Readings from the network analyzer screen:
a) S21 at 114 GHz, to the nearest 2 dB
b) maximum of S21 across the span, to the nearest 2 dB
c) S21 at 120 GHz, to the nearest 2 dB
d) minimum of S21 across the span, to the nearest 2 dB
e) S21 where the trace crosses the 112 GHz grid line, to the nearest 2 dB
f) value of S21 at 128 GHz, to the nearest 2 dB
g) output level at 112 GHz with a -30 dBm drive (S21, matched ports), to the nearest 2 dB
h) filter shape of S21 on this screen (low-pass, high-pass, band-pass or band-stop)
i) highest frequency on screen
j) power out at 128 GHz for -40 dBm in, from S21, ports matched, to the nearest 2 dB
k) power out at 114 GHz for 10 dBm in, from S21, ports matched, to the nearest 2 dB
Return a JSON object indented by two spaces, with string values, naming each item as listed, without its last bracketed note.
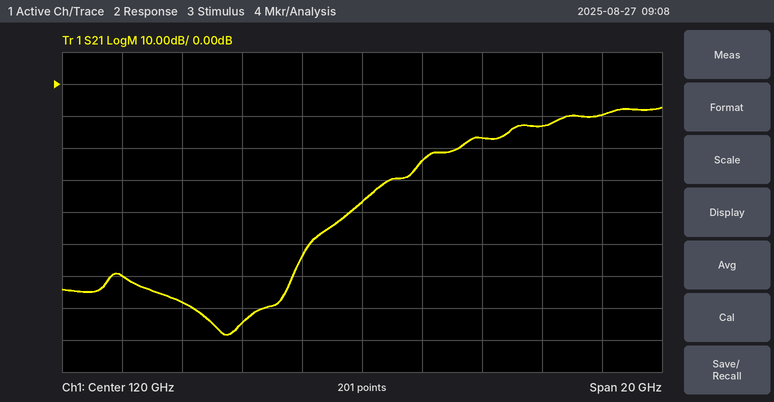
{
  "S21 at 114 GHz, to the nearest 2 dB": "-68 dB",
  "maximum of S21 across the span, to the nearest 2 dB": "-8 dB",
  "S21 at 120 GHz, to the nearest 2 dB": "-36 dB",
  "minimum of S21 across the span, to the nearest 2 dB": "-78 dB",
  "S21 where the trace crosses the 112 GHz grid line, to the nearest 2 dB": "-60 dB",
  "value of S21 at 128 GHz, to the nearest 2 dB": "-10 dB",
  "output level at 112 GHz with a -30 dBm drive (S21, matched ports), to the nearest 2 dB": "-90 dBm",
  "filter shape of S21 on this screen": "high-pass",
  "highest frequency on screen": "130 GHz",
  "power out at 128 GHz for -40 dBm in, from S21, ports matched, to the nearest 2 dB": "-50 dBm",
  "power out at 114 GHz for 10 dBm in, from S21, ports matched, to the nearest 2 dB": "-58 dBm"
}
